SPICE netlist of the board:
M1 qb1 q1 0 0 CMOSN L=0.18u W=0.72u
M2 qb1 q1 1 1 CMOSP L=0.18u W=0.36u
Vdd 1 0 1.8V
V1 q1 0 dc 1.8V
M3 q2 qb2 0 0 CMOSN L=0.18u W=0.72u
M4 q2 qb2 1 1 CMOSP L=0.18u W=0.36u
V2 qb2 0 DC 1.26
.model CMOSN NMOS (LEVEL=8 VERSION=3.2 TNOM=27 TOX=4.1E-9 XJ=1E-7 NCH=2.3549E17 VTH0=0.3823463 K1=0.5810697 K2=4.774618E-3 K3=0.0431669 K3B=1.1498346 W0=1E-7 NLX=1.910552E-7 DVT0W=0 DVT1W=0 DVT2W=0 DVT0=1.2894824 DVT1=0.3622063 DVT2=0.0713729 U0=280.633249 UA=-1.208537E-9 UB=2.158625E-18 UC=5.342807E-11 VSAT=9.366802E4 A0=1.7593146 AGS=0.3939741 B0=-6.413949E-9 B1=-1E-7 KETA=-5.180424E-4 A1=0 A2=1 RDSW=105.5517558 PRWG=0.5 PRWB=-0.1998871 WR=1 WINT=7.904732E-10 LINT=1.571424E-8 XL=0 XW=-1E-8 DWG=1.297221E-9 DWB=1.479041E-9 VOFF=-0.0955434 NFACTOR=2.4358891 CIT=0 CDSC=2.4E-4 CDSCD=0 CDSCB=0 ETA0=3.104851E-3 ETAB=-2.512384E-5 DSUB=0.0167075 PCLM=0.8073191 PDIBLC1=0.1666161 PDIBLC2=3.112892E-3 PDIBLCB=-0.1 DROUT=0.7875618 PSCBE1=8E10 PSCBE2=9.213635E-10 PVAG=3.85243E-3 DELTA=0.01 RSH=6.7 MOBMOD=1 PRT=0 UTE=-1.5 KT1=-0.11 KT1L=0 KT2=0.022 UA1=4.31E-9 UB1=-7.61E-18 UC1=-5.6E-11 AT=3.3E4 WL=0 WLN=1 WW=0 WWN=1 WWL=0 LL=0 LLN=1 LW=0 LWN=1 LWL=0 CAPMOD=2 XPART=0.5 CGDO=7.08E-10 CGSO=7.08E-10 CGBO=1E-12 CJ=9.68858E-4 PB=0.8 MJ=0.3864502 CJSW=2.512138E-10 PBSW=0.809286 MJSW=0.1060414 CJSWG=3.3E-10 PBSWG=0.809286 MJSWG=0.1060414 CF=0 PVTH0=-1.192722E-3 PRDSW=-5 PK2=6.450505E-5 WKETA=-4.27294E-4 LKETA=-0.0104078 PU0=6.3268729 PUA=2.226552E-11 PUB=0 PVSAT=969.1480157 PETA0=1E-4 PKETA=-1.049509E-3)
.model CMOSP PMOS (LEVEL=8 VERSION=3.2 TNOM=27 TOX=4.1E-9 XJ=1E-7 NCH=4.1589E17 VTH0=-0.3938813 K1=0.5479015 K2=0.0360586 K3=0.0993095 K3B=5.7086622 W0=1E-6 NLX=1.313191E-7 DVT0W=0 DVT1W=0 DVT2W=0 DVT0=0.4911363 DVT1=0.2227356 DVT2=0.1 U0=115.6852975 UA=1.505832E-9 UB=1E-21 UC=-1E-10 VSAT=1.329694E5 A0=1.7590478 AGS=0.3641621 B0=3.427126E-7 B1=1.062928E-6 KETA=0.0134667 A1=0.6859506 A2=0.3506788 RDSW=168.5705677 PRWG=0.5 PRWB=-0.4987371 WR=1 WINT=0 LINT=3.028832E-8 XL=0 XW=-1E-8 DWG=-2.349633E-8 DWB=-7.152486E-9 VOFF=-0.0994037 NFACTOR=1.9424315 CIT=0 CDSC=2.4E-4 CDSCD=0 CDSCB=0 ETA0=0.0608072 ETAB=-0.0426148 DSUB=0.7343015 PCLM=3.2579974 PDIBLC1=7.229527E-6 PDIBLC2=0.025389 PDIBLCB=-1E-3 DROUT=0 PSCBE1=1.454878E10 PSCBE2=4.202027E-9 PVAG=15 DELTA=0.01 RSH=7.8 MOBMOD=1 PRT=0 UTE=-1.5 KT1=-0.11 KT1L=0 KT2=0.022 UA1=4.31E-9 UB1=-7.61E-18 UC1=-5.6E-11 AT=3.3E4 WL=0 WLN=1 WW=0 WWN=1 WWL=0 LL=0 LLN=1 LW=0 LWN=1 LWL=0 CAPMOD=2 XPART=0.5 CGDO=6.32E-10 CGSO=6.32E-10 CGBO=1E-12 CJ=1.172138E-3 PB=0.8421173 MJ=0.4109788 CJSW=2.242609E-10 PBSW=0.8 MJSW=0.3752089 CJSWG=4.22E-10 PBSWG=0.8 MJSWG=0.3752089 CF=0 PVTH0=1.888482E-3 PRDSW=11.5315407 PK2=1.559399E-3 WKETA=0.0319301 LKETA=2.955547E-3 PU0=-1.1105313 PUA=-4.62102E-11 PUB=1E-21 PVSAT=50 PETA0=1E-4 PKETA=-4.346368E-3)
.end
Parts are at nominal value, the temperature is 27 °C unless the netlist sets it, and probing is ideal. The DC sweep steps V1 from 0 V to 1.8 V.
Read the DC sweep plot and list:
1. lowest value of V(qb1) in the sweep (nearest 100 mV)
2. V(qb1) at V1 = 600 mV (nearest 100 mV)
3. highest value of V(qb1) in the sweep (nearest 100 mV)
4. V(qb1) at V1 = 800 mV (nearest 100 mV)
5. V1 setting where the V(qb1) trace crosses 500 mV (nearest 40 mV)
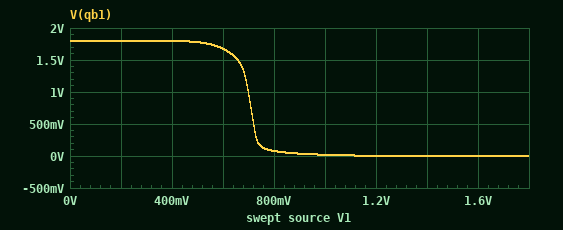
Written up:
0 V
1.7 V
1.8 V
100 mV
720 mV
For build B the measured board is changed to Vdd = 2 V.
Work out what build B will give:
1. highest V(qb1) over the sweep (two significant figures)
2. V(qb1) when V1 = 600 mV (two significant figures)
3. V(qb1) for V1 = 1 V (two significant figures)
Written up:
2.0 V
1.9 V
43 mV
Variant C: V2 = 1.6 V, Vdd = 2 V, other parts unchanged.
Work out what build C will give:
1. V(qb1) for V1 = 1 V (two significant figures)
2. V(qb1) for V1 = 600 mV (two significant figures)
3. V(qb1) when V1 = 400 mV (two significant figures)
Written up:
43 mV
1.9 V
2.0 V
